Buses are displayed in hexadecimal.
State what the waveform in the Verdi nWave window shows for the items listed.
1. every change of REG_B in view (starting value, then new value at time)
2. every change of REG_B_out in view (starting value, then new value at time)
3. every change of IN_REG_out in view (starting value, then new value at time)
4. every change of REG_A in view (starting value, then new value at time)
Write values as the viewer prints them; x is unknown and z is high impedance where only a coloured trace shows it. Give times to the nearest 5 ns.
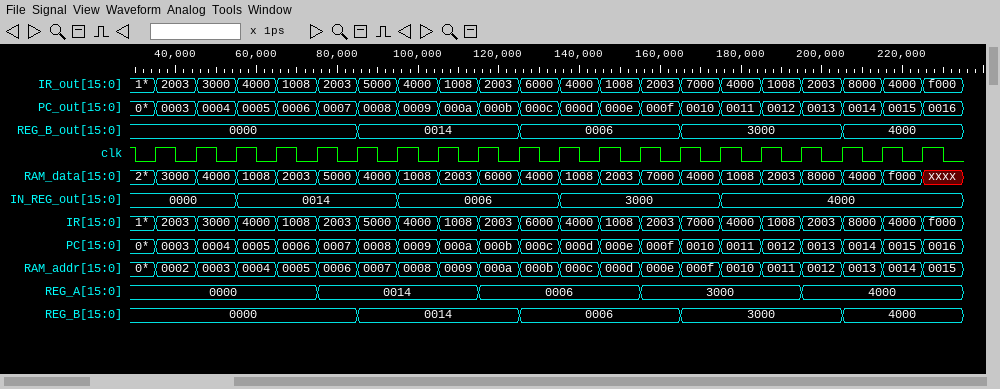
0000, 0014 at 85 ns, 0006 at 125 ns, 3000 at 165 ns, 4000 at 205 ns
0000, 0014 at 85 ns, 0006 at 125 ns, 3000 at 165 ns, 4000 at 205 ns
0000, 0014 at 55 ns, 0006 at 95 ns, 3000 at 135 ns, 4000 at 175 ns
0000, 0014 at 75 ns, 0006 at 115 ns, 3000 at 155 ns, 4000 at 195 ns
